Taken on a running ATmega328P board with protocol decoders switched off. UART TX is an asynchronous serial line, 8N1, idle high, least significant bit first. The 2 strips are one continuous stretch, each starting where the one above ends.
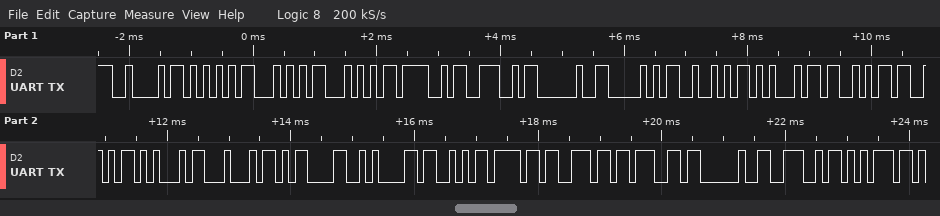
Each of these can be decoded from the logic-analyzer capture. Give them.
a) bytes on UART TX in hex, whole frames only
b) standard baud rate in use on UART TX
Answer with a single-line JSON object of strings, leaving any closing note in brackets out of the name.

{"bytes on UART TX in hex, whole frames only": "42 55 54 54 4F 4E 20 50 52 45 53 53 45 44 0D 0A 53 6F 6E 67 20 4E 75", "standard baud rate in use on UART TX": "9600 baud"}
